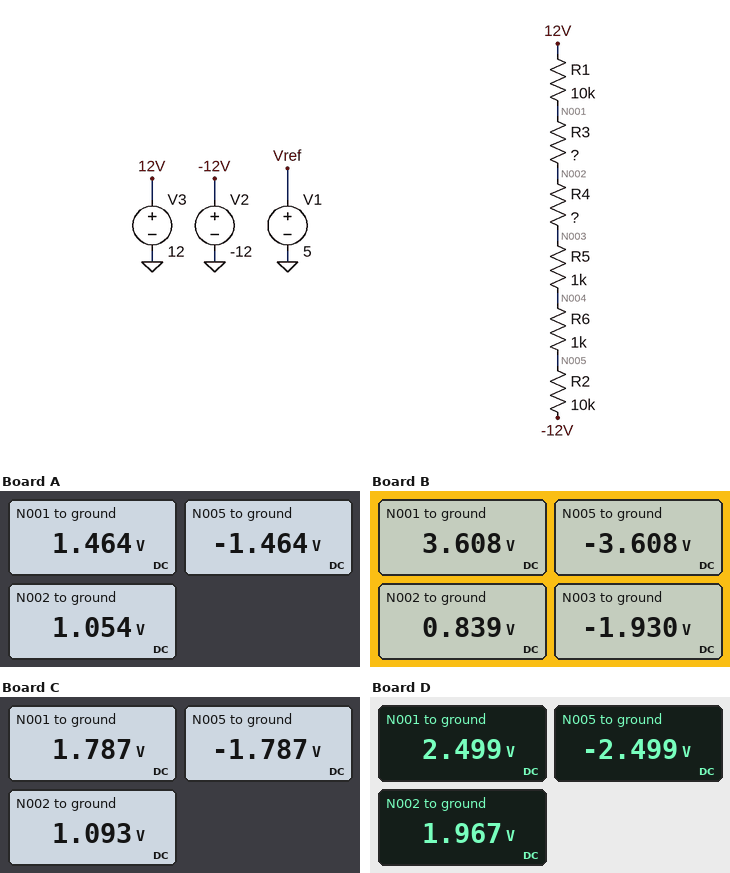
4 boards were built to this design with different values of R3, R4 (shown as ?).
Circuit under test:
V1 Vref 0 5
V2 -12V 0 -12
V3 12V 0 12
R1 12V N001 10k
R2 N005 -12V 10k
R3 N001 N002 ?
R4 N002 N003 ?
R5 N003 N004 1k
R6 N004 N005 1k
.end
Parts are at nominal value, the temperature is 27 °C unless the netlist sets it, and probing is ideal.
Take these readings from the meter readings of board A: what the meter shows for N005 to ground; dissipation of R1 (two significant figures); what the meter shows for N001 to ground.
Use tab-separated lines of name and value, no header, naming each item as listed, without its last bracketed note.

what the meter shows for N005 to ground	-1.464 V
dissipation of R1	11 mW
what the meter shows for N001 to ground	1.464 V
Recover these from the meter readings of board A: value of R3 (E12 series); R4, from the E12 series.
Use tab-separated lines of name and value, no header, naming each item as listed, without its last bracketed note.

value of R3	390 Ω
R4, from the E12 series	390 Ω
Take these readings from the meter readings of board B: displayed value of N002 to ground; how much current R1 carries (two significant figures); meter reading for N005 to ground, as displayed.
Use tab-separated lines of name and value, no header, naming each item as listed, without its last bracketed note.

displayed value of N002 to ground	0.839 V
how much current R1 carries	840 µA
meter reading for N005 to ground, as displayed	-3.608 V
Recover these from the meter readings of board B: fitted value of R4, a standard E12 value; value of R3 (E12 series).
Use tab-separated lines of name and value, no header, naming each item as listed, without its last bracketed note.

fitted value of R4, a standard E12 value	3.3 kΩ
value of R3	3.3 kΩ
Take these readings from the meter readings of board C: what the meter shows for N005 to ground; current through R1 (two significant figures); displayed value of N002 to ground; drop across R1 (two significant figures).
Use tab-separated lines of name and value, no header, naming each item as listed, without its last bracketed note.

what the meter shows for N005 to ground	-1.787 V
current through R1	1.0 mA
displayed value of N002 to ground	1.093 V
drop across R1	10 V
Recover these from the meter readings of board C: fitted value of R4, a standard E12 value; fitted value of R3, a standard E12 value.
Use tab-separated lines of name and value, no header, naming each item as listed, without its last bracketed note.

fitted value of R4, a standard E12 value	820 Ω
fitted value of R3, a standard E12 value	680 Ω
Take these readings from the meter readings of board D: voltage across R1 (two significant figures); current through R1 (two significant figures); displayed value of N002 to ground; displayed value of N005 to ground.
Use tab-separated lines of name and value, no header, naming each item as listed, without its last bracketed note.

voltage across R1	9.5 V
current through R1	950 µA
displayed value of N002 to ground	1.967 V
displayed value of N005 to ground	-2.499 V
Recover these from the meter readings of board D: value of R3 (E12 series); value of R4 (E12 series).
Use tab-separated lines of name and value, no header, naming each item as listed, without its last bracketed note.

value of R3	560 Ω
value of R4	2.7 kΩ
